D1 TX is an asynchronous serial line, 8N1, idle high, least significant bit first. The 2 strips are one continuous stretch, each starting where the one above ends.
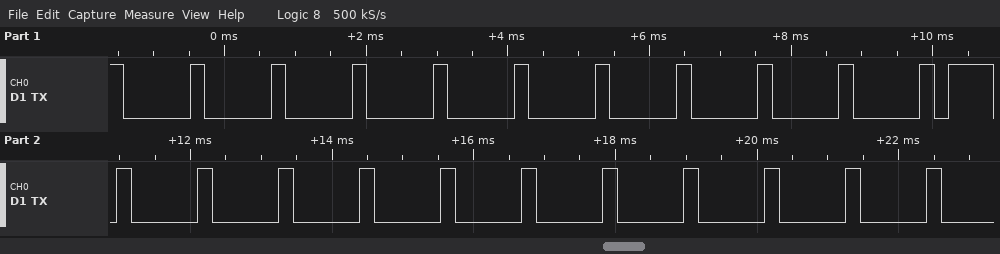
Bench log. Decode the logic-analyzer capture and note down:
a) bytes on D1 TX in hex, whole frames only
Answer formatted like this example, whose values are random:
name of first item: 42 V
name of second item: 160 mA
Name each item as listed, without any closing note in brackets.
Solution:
bytes on D1 TX in hex, whole frames only: 00 00 00 00 00 00 00 00 00 00 7E 00 00 00 00 00 00 00 00 00 00
